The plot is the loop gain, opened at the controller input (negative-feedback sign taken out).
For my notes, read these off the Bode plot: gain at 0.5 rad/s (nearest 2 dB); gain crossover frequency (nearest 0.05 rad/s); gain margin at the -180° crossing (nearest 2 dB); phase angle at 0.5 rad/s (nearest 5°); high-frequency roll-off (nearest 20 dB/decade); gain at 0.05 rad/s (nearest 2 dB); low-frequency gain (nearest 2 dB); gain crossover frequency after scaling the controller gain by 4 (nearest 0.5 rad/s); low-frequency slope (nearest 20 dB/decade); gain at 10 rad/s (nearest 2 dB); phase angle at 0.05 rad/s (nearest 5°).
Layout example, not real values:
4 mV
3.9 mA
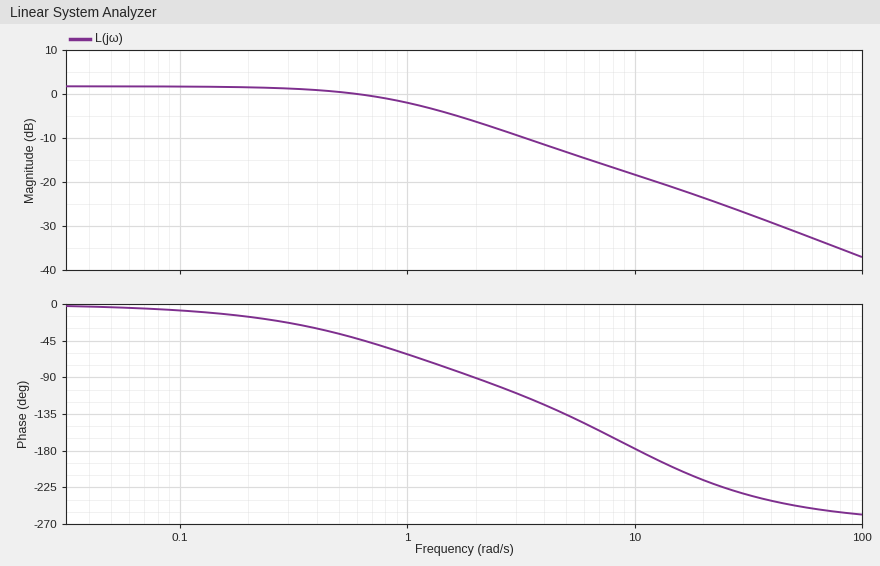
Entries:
0 dB
0.60 rad/s
18 dB
-35°
-20 dB/decade
2 dB
2 dB
4.5 rad/s
0 dB/decade
-18 dB
-5°
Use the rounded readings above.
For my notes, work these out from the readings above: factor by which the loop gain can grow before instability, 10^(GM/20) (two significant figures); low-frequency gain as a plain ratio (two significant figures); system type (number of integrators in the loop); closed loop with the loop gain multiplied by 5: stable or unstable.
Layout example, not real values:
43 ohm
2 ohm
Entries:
7.9
1.3
0
stable
